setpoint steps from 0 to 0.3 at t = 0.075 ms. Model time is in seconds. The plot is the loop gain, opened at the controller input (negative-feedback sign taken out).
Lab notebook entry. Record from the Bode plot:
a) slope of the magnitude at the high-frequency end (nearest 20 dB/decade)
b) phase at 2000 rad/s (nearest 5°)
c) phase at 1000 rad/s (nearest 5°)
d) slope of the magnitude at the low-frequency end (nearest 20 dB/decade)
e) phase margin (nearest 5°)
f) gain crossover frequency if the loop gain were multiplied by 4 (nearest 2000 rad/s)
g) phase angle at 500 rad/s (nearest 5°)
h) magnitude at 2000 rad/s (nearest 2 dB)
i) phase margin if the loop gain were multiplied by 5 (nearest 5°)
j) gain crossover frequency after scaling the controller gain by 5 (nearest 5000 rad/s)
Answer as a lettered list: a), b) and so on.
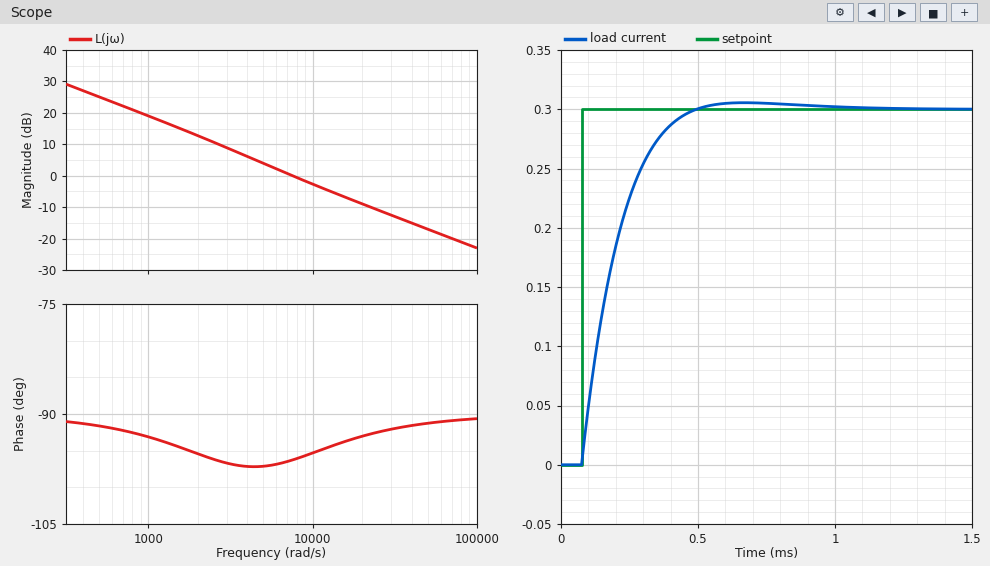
a) -20 dB/decade
b) -95°
c) -95°
d) -20 dB/decade
e) 85°
f) 28000 rad/s
g) -90°
h) 12 dB
i) 90°
j) 35000 rad/s
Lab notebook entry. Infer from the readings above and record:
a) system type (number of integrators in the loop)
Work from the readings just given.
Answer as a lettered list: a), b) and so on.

a) 1
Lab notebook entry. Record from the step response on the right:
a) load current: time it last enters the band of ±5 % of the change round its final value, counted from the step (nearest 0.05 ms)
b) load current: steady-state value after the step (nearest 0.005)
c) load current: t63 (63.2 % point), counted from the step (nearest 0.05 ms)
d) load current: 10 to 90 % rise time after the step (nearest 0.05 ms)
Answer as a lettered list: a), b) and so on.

a) 0.30 ms
b) 0.300
c) 0.15 ms
d) 0.25 ms
